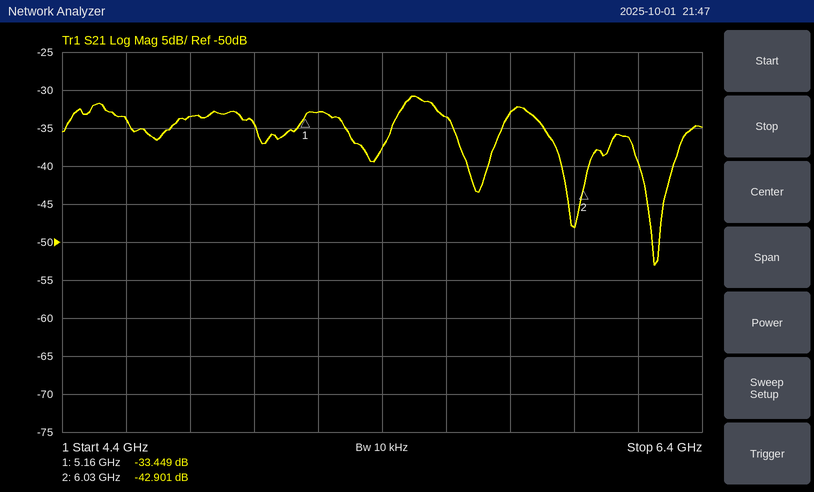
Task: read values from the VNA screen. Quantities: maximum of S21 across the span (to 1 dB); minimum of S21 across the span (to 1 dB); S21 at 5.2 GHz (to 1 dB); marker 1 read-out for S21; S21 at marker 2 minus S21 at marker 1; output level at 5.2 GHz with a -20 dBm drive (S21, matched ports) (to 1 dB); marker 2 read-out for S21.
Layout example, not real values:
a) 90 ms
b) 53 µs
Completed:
a) -31 dB
b) -53 dB
c) -33 dB
d) -33.449 dB
e) -9.452 dB
f) -53 dBm
g) -42.901 dB
